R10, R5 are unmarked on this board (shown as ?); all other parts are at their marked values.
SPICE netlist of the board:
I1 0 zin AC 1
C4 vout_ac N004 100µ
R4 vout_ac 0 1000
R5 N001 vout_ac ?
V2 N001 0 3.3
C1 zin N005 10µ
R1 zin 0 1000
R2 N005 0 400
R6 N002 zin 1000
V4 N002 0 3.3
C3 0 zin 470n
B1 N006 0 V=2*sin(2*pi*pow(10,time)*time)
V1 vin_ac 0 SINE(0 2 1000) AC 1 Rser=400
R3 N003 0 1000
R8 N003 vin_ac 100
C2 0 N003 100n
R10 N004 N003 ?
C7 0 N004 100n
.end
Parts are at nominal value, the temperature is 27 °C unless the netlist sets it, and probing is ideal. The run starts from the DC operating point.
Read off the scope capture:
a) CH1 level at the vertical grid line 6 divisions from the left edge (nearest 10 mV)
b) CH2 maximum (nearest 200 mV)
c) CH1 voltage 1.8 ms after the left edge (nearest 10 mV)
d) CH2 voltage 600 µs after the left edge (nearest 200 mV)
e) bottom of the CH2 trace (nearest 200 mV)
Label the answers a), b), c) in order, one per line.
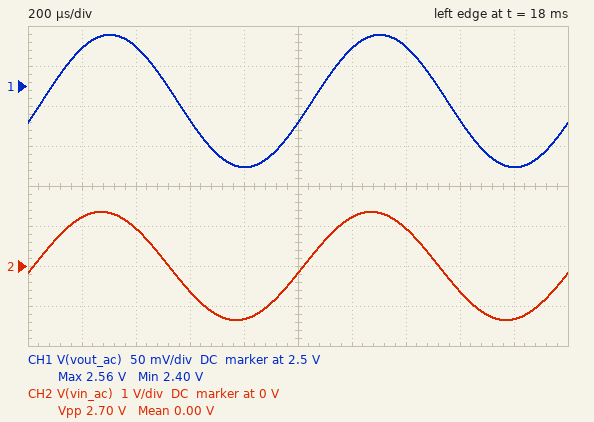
a) 2.55 V
b) 1.4 V
c) 2.40 V
d) -600 mV
e) -1.4 V
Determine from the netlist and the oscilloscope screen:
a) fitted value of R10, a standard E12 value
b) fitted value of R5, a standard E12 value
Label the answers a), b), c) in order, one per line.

a) 3.3 kΩ
b) 330 Ω
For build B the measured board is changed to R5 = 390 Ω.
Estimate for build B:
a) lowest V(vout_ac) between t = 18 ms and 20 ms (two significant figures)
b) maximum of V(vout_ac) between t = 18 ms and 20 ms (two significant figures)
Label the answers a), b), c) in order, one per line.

a) 2.3 V
b) 2.5 V
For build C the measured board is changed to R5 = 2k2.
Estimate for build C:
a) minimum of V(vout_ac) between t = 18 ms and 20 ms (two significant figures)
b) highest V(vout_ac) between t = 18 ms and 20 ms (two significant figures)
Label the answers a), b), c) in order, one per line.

a) 840 mV
b) 1.2 V
